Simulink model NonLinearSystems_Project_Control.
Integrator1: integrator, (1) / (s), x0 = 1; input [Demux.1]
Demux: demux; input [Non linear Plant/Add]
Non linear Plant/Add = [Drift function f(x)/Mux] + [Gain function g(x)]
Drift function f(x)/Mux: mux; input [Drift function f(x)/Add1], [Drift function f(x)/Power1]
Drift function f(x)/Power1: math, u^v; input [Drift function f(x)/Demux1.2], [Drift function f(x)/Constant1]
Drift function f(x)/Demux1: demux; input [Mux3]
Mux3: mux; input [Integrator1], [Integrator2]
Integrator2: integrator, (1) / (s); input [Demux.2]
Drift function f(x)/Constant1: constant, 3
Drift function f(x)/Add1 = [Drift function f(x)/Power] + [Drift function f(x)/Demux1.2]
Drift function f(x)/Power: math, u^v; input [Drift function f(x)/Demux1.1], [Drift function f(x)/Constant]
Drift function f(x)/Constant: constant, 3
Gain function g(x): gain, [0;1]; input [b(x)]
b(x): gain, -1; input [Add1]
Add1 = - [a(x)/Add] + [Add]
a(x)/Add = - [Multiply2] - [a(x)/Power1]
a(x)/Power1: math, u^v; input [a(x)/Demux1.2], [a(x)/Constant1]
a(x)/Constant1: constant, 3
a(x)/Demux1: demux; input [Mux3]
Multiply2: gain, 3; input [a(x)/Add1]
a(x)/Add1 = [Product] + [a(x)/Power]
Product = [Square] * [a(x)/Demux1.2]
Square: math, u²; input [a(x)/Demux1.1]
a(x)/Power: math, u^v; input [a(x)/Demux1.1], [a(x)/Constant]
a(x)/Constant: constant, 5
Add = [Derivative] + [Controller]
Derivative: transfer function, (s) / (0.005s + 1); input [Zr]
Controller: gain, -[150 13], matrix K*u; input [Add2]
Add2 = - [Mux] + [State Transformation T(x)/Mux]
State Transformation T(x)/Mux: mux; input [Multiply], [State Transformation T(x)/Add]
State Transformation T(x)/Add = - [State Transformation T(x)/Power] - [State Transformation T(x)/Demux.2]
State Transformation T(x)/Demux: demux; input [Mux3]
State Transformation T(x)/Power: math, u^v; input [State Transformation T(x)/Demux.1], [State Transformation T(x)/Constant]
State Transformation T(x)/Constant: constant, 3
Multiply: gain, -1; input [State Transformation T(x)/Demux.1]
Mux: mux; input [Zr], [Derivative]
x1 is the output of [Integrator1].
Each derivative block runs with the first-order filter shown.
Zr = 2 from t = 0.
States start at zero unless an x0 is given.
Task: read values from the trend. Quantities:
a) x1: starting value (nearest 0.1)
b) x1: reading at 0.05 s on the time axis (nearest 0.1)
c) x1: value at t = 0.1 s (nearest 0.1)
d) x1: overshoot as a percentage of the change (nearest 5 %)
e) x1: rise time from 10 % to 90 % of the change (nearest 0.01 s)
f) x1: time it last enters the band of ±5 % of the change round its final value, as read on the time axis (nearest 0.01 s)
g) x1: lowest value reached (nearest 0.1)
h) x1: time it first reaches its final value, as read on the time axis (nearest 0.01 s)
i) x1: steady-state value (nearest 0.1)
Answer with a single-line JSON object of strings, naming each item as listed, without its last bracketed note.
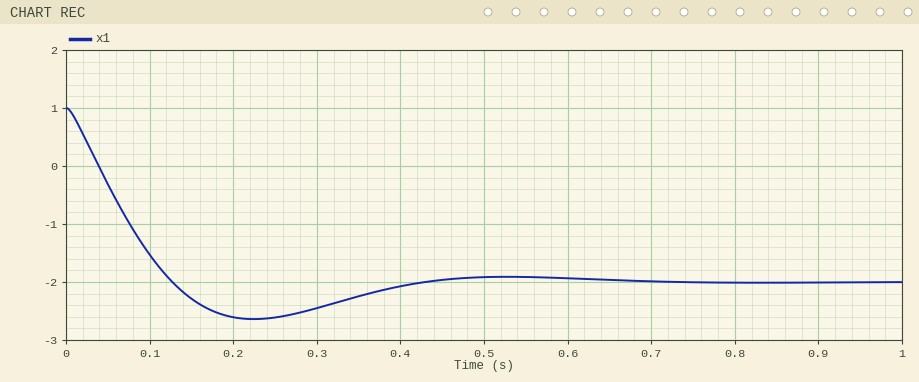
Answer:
{"x1: starting value": "1.0", "x1: reading at 0.05 s on the time axis": "-0.3", "x1: value at t = 0.1 s": "-1.5", "x1: overshoot as a percentage of the change": "20 %", "x1: rise time from 10 % to 90 % of the change": "0.09 s", "x1: time it last enters the band of ±5 % of the change round its final value, as read on the time axis": "0.38 s", "x1: lowest value reached": "-2.6", "x1: time it first reaches its final value, as read on the time axis": "0.13 s", "x1: steady-state value": "-2.0"}
